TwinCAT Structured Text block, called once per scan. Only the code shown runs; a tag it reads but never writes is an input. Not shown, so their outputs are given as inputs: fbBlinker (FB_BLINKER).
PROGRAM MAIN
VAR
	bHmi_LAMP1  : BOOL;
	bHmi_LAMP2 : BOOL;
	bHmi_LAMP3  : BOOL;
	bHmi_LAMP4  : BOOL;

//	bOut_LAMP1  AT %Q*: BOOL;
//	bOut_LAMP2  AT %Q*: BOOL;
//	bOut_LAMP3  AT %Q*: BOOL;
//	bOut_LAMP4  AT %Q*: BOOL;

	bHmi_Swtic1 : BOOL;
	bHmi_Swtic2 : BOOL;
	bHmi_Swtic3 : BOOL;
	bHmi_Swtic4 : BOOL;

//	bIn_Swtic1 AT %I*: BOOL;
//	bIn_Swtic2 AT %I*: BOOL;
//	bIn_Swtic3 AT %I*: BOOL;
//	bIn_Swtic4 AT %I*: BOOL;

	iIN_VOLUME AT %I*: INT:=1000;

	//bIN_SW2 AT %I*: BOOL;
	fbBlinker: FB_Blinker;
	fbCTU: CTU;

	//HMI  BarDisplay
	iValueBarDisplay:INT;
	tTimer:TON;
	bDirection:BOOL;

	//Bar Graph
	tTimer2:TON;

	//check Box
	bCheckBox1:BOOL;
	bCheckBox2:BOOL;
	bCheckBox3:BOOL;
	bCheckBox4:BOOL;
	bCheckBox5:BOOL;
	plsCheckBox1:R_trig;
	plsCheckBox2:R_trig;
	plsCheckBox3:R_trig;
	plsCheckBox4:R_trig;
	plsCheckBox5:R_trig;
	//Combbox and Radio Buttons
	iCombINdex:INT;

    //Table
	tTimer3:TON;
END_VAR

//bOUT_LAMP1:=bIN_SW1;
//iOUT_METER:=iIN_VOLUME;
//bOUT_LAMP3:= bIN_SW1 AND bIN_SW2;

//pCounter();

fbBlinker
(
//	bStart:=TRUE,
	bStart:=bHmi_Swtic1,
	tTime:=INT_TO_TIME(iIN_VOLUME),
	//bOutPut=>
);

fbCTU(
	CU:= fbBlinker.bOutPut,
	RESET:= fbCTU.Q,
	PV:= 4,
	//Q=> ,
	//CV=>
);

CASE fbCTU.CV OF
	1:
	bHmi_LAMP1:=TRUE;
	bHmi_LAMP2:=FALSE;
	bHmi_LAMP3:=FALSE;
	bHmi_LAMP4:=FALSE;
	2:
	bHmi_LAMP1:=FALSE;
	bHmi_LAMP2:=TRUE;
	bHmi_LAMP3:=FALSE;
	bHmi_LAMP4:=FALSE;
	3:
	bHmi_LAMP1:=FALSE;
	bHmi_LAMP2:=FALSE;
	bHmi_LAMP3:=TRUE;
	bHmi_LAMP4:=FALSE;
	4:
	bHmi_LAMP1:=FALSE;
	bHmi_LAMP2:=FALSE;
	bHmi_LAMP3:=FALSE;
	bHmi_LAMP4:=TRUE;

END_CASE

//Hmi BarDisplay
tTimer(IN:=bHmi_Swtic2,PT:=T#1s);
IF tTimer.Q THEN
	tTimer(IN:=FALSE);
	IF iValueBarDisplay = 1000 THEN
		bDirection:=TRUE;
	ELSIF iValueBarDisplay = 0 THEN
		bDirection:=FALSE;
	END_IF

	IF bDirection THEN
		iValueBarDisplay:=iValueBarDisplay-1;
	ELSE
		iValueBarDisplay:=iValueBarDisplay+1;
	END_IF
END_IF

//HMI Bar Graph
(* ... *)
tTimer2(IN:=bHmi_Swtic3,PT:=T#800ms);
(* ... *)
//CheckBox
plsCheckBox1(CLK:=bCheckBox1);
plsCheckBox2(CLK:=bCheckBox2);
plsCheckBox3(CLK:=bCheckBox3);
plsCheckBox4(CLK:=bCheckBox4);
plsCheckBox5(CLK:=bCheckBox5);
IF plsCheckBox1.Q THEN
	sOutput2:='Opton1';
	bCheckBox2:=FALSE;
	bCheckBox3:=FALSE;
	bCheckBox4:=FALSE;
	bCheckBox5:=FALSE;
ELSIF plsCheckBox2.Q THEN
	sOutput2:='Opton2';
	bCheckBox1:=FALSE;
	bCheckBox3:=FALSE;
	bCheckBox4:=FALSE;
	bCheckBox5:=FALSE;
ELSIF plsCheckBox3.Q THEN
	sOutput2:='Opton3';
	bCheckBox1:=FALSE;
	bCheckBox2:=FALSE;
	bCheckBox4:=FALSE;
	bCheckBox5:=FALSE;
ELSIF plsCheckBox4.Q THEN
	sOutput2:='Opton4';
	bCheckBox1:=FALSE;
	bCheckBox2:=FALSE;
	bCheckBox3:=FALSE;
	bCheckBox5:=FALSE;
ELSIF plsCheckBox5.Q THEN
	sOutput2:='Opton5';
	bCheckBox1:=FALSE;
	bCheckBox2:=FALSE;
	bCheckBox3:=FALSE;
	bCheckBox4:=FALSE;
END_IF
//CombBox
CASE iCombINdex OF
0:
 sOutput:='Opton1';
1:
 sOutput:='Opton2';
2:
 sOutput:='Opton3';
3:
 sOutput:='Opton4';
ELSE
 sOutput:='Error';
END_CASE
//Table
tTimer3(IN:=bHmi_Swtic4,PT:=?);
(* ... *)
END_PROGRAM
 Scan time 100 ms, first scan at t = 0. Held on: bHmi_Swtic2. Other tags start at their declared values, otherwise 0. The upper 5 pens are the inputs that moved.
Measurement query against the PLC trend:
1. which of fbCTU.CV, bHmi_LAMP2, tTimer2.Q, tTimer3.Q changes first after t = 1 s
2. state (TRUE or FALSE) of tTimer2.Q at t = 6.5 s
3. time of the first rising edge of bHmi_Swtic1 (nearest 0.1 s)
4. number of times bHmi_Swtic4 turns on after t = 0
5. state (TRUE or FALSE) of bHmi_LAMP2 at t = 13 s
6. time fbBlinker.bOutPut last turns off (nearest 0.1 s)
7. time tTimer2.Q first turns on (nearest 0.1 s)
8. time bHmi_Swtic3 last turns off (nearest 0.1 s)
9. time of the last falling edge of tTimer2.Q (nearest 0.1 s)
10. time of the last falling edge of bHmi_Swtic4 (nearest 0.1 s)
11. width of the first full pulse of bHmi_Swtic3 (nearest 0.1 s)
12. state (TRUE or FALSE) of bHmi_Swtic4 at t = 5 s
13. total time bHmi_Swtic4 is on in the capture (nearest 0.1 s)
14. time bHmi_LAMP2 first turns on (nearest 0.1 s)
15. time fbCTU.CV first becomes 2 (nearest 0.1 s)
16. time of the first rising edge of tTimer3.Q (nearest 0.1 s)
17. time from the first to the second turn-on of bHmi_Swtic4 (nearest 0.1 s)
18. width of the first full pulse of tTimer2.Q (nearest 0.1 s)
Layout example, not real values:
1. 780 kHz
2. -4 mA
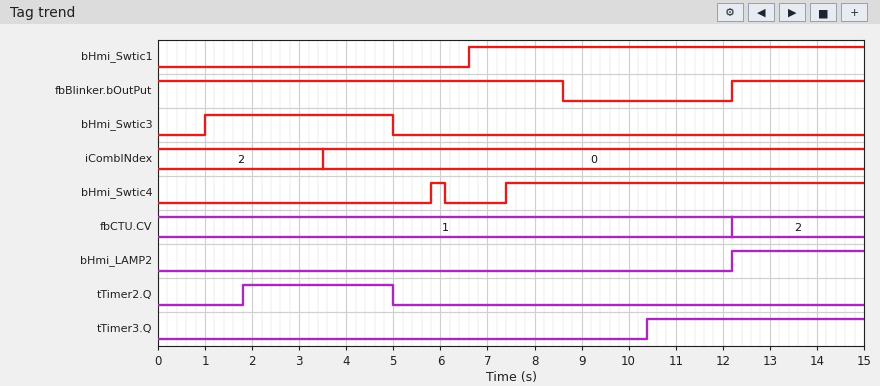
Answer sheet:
1. tTimer2.Q
2. FALSE
3. 6.6 s
4. 2
5. TRUE
6. 8.6 s
7. 1.8 s
8. 5.0 s
9. 5.0 s
10. 6.1 s
11. 4.0 s
12. FALSE
13. 7.9 s
14. 12.2 s
15. 12.2 s
16. 10.4 s
17. 1.6 s
18. 3.2 s
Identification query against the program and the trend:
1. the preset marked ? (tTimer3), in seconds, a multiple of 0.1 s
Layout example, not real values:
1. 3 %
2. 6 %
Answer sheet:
1. 3.0 s
